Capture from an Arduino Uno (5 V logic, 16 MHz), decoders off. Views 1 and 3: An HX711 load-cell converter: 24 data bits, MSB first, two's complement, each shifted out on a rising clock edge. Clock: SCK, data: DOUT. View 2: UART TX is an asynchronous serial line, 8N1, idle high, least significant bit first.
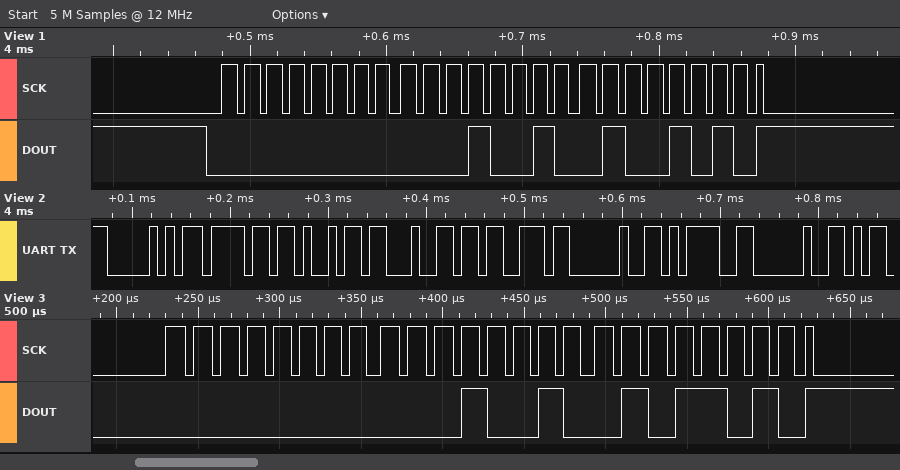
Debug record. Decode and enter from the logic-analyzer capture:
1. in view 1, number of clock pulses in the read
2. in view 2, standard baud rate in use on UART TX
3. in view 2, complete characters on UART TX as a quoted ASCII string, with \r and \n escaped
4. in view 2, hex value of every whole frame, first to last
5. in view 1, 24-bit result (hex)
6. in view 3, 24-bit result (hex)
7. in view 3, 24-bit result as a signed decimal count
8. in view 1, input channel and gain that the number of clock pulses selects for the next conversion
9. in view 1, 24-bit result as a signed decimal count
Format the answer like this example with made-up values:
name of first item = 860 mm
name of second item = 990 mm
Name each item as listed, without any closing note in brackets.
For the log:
in view 1, number of clock pulses in the read = 25
in view 2, standard baud rate in use on UART TX = 115200 baud
in view 2, complete characters on UART TX as a quoted ASCII string, with \r and \n escaped = "Poids = "
in view 2, hex value of every whole frame, first to last = 50 6F 69 64 73 20 3D 20
in view 1, 24-bit result = 0x00124A
in view 3, 24-bit result = 0x00125A
in view 3, 24-bit result as a signed decimal count = 4698
in view 1, input channel and gain that the number of clock pulses selects for the next conversion = channel A, gain 128
in view 1, 24-bit result as a signed decimal count = 4682
